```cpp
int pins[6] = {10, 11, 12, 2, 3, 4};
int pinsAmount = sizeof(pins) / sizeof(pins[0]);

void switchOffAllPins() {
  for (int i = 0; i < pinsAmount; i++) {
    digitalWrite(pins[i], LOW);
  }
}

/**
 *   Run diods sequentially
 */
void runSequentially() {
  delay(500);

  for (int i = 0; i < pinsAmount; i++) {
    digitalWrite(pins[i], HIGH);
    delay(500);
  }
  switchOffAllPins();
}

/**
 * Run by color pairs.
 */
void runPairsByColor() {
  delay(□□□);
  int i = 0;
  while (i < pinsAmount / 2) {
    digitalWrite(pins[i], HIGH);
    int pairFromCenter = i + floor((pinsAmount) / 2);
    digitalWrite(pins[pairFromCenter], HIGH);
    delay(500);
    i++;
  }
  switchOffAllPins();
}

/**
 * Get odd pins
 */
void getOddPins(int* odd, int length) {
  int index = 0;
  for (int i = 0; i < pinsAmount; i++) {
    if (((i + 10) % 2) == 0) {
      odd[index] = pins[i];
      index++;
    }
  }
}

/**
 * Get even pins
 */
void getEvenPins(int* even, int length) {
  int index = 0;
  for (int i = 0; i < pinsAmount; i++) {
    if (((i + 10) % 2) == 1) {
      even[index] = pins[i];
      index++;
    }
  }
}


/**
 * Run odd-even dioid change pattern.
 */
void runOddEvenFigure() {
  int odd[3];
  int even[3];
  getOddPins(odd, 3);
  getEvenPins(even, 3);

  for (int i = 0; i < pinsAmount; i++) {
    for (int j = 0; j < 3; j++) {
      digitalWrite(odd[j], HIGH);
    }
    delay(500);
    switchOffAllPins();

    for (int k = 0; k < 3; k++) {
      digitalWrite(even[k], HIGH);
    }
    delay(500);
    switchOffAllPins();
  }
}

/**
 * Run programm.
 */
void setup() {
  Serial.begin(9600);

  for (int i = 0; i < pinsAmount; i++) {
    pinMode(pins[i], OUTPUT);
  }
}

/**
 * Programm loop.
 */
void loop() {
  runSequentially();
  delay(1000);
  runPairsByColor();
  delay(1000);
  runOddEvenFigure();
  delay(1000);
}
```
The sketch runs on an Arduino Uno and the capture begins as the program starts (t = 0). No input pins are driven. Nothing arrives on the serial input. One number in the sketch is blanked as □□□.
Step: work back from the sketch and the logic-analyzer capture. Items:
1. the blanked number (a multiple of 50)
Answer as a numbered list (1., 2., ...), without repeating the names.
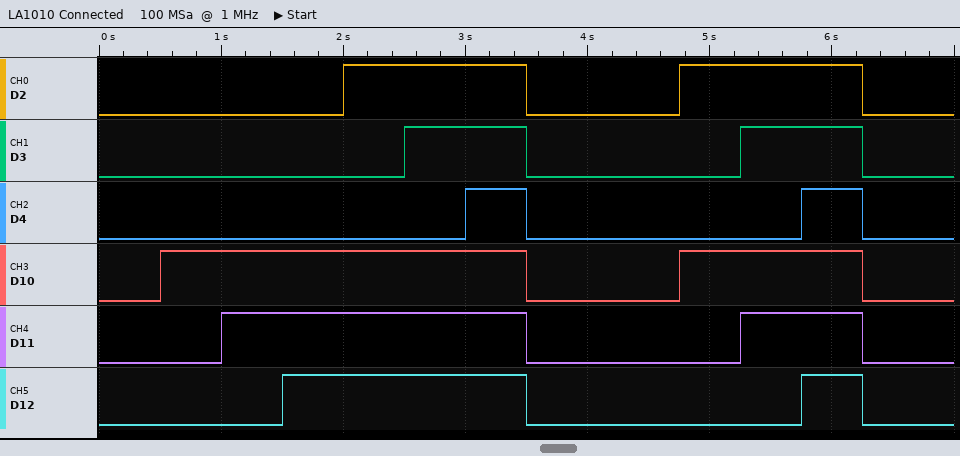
1. 250
